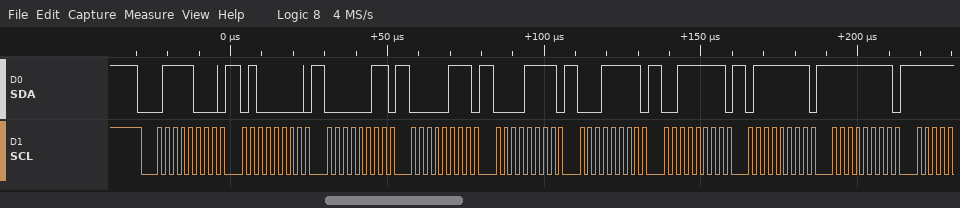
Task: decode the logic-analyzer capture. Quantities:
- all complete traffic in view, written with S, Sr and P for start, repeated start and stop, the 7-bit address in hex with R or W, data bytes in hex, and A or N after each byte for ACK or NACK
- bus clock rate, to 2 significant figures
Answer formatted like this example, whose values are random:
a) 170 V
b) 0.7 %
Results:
a) S 3CW A 40 A 03 A 07 A 0F A 1F A 3F A 7F A FF A
b) 400 kHz
